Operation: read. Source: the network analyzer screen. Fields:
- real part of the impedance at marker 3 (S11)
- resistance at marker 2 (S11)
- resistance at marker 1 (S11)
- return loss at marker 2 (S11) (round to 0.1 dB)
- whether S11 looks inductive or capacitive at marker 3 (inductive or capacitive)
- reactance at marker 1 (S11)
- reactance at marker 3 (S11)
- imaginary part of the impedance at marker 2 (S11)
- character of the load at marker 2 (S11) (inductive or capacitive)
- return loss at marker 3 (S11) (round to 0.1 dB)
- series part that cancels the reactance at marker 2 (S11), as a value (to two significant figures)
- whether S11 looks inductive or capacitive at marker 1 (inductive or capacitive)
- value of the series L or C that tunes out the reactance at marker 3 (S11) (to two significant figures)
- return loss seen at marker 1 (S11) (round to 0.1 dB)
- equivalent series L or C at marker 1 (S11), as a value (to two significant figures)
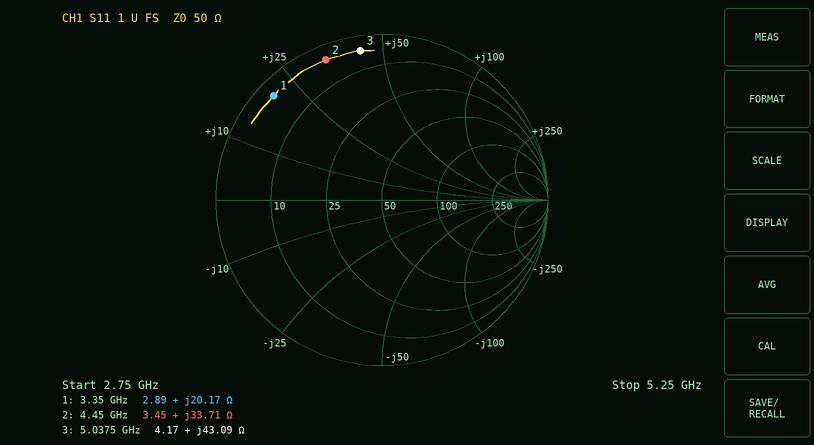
4.17 Ω
3.45 Ω
2.89 Ω
0.8 dB
inductive
+20.17 Ω
+43.09 Ω
+33.71 Ω
inductive
0.8 dB
1.1 pF
inductive
730 fF
0.9 dB
960 pH
